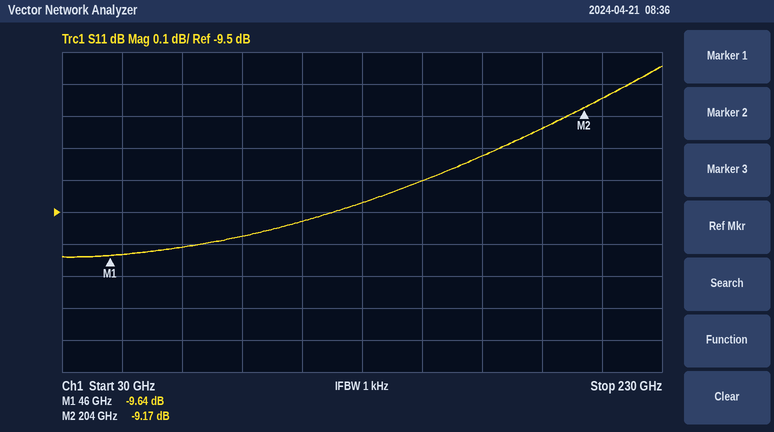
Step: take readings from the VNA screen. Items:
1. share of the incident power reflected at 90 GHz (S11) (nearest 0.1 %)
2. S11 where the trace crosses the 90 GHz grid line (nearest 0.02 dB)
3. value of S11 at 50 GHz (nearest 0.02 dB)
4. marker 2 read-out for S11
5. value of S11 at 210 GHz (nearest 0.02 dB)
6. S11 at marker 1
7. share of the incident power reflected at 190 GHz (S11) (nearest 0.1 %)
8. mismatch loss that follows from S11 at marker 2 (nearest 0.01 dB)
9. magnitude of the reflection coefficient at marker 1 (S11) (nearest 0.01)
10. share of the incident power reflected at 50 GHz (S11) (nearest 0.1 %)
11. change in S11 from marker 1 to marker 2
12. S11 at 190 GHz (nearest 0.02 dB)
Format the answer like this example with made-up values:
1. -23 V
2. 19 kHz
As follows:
1. 11.0 %
2. -9.58 dB
3. -9.64 dB
4. -9.17 dB
5. -9.14 dB
6. -9.64 dB
7. 11.9 %
8. 0.56 dB
9. 0.33
10. 10.9 %
11. 0.47 dB
12. -9.24 dB
